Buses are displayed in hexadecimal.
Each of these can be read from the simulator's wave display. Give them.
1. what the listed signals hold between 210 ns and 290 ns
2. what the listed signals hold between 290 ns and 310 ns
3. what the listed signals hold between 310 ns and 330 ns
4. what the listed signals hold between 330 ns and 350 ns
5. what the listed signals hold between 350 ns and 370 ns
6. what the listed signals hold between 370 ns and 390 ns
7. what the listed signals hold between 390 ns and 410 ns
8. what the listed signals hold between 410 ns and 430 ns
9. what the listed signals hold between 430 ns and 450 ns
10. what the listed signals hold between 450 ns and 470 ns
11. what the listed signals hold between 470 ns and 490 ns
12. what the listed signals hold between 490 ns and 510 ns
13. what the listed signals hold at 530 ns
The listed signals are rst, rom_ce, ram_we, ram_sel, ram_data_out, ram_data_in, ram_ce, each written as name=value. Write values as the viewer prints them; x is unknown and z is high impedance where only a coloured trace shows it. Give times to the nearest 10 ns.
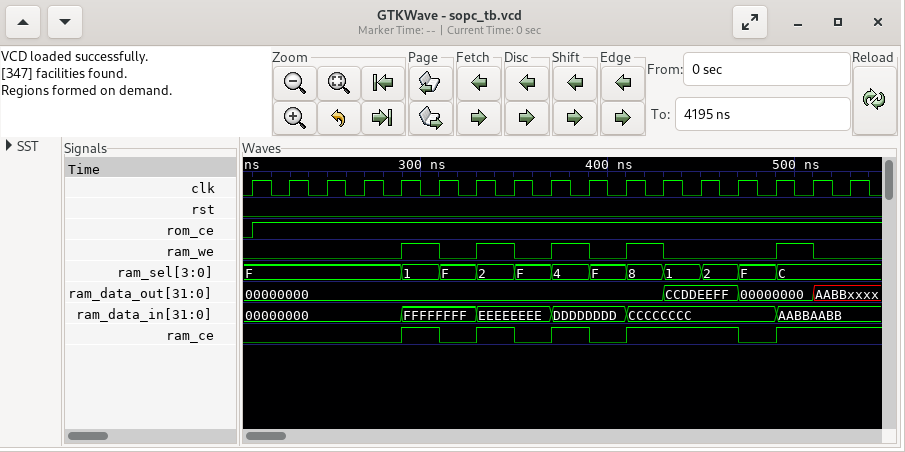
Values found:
rst=0, rom_ce=1, ram_we=0, ram_sel=F, ram_data_out=00000000, ram_data_in=00000000, ram_ce=0
rst=0, rom_ce=1, ram_we=1, ram_sel=1, ram_data_out=00000000, ram_data_in=FFFFFFFF, ram_ce=1
rst=0, rom_ce=1, ram_we=0, ram_sel=F, ram_data_out=00000000, ram_data_in=FFFFFFFF, ram_ce=0
rst=0, rom_ce=1, ram_we=1, ram_sel=2, ram_data_out=00000000, ram_data_in=EEEEEEEE, ram_ce=1
rst=0, rom_ce=1, ram_we=0, ram_sel=F, ram_data_out=00000000, ram_data_in=EEEEEEEE, ram_ce=0
rst=0, rom_ce=1, ram_we=1, ram_sel=4, ram_data_out=00000000, ram_data_in=DDDDDDDD, ram_ce=1
rst=0, rom_ce=1, ram_we=0, ram_sel=F, ram_data_out=00000000, ram_data_in=DDDDDDDD, ram_ce=0
rst=0, rom_ce=1, ram_we=1, ram_sel=8, ram_data_out=00000000, ram_data_in=CCCCCCCC, ram_ce=1
rst=0, rom_ce=1, ram_we=0, ram_sel=1, ram_data_out=CCDDEEFF, ram_data_in=CCCCCCCC, ram_ce=1
rst=0, rom_ce=1, ram_we=0, ram_sel=2, ram_data_out=CCDDEEFF, ram_data_in=CCCCCCCC, ram_ce=1
rst=0, rom_ce=1, ram_we=0, ram_sel=F, ram_data_out=00000000, ram_data_in=CCCCCCCC, ram_ce=0
rst=0, rom_ce=1, ram_we=1, ram_sel=C, ram_data_out=00000000, ram_data_in=AABBAABB, ram_ce=1
rst=0, rom_ce=1, ram_we=0, ram_sel=C, ram_data_out=AABBxxxx, ram_data_in=AABBAABB, ram_ce=1
